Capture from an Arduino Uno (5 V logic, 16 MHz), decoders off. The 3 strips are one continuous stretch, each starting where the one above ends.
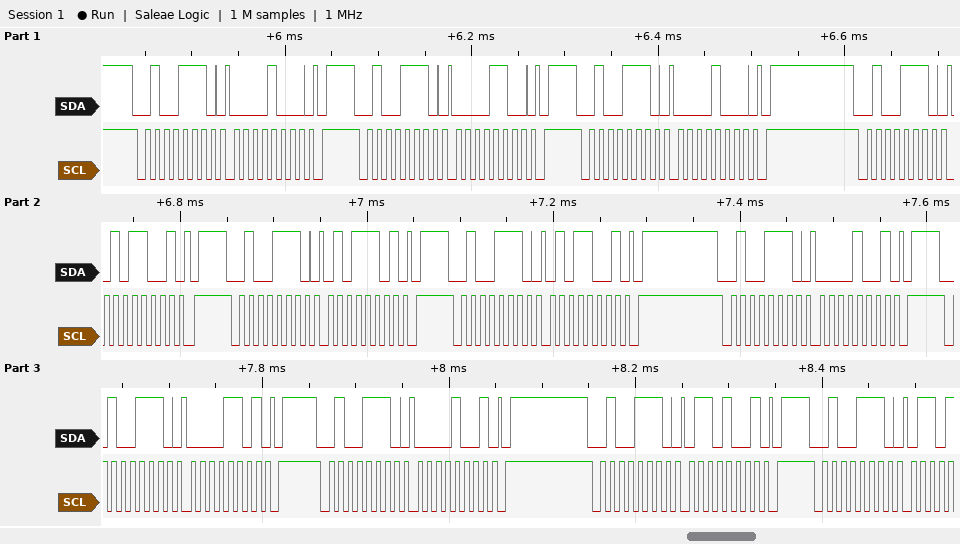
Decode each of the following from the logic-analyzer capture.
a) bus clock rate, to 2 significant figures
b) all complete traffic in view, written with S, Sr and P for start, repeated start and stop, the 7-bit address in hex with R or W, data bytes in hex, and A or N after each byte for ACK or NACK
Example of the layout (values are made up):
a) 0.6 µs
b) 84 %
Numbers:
a) 100 kHz
b) S 27W A 08 A P S 27W A 0C A P S 27W A 08 A P S 27W A 59 A P S 27W A 5D A P S 27W A 59 A P S 27W A 09 A P S 27W A 0D A P S 27W A 09 A P S 27W A 69 A P S 27W A
